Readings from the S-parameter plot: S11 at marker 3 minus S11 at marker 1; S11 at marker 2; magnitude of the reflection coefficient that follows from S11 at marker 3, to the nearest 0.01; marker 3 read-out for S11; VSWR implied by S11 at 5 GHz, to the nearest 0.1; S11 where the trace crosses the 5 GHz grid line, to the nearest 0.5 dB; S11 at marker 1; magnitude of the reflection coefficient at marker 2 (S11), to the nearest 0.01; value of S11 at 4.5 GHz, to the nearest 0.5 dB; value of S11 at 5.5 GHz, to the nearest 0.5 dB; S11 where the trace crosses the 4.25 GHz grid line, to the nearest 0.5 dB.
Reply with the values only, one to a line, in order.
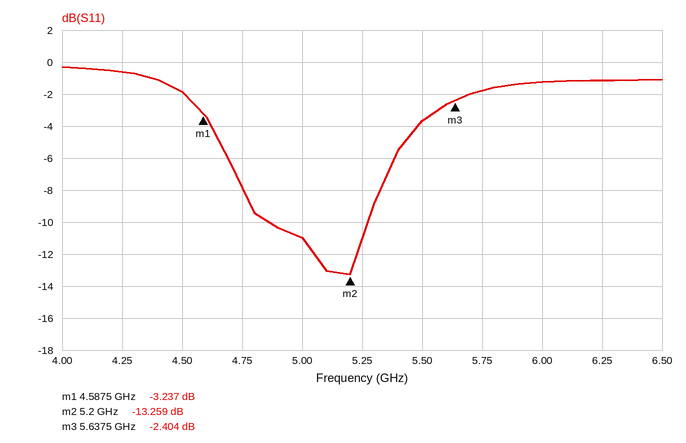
0.833 dB
-13.259 dB
0.76
-2.404 dB
1.8
-11.0 dB
-3.237 dB
0.22
-2.0 dB
-3.5 dB
-0.5 dB
